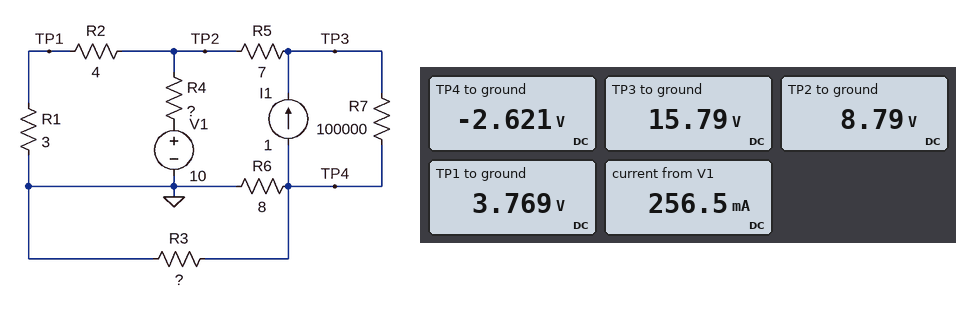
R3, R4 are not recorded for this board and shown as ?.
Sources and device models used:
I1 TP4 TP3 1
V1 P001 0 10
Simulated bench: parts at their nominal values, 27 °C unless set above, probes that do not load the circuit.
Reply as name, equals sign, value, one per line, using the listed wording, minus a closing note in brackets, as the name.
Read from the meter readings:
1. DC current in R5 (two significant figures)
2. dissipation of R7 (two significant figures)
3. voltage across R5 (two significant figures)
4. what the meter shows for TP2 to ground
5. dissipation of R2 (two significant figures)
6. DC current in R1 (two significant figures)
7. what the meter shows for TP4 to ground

DC current in R5 = 1.0 A
dissipation of R7 = 3.4 mW
voltage across R5 = 7.0 V
what the meter shows for TP2 to ground = 8.79 V
dissipation of R2 = 6.3 W
DC current in R1 = 1.3 A
what the meter shows for TP4 to ground = -2.621 V
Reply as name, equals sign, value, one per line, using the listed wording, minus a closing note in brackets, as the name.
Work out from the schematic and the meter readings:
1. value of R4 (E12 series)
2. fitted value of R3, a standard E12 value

value of R4 = 4.7 Ω
fitted value of R3, a standard E12 value = 3.9 Ω
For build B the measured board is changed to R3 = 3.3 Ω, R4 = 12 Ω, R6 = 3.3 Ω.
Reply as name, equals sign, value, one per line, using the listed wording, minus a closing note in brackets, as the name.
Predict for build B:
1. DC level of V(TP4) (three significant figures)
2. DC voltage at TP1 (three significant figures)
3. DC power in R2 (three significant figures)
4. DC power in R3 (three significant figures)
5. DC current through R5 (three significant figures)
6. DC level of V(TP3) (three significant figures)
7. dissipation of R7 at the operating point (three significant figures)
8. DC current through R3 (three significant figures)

DC level of V(TP4) = -1.65 V
DC voltage at TP1 = 3.47 V
DC power in R2 = 5.36 W
DC power in R3 = 825 mW
DC current through R5 = 1.00 A
DC level of V(TP3) = 15.1 V
dissipation of R7 at the operating point = 2.81 mW
DC current through R3 = 500 mA
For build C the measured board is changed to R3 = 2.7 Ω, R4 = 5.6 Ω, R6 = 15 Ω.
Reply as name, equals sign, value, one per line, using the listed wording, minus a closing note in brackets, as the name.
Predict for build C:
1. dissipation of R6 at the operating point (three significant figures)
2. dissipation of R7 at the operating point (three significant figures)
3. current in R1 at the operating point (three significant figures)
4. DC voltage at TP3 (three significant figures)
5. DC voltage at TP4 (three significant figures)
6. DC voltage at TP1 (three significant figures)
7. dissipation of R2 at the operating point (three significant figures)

dissipation of R6 at the operating point = 349 mW
dissipation of R7 at the operating point = 3.22 mW
current in R1 at the operating point = 1.24 A
DC voltage at TP3 = 15.7 V
DC voltage at TP4 = -2.29 V
DC voltage at TP1 = 3.71 V
dissipation of R2 at the operating point = 6.13 W
